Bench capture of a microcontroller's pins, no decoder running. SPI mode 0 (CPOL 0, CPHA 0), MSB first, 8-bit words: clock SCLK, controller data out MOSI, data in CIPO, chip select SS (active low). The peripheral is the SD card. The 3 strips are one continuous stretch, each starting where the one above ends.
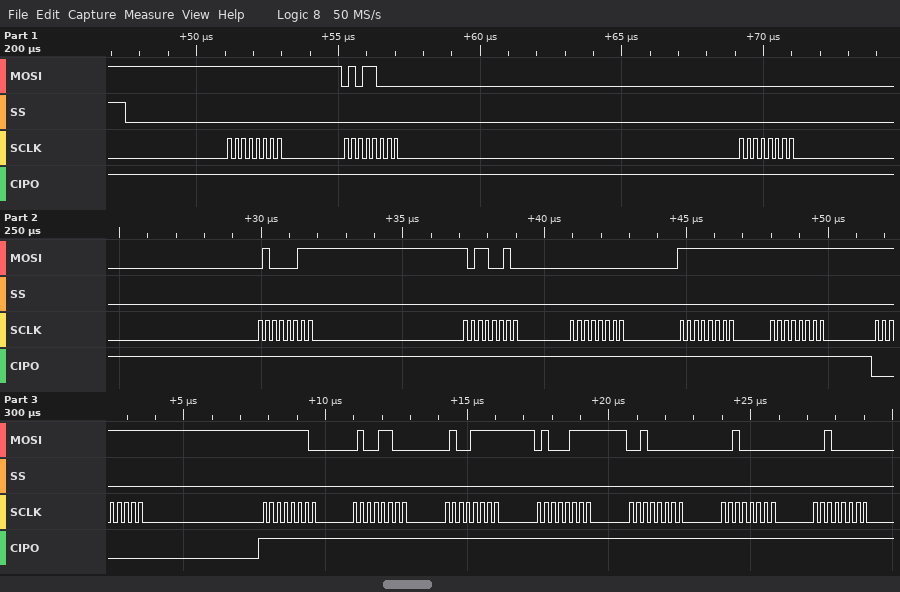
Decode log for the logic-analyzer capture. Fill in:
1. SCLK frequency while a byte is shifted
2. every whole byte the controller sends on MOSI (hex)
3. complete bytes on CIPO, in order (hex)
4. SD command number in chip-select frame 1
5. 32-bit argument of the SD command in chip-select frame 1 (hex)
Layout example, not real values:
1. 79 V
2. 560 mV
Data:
1. 4 MHz
2. FF 58 00 43 B2 00 FF FF FF FE 4C 4F 47 20 20 20
3. FF FF FF FF FF FF FF FF 00 FF FF FF FF FF FF FF
4. CMD24
5. 0x0043B200
